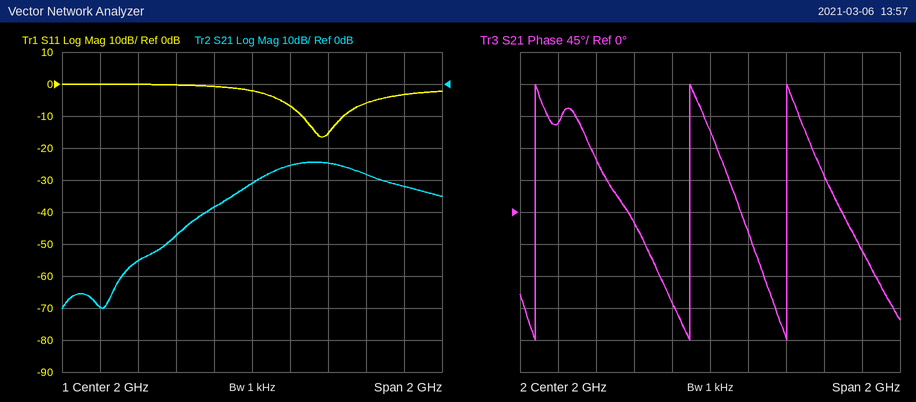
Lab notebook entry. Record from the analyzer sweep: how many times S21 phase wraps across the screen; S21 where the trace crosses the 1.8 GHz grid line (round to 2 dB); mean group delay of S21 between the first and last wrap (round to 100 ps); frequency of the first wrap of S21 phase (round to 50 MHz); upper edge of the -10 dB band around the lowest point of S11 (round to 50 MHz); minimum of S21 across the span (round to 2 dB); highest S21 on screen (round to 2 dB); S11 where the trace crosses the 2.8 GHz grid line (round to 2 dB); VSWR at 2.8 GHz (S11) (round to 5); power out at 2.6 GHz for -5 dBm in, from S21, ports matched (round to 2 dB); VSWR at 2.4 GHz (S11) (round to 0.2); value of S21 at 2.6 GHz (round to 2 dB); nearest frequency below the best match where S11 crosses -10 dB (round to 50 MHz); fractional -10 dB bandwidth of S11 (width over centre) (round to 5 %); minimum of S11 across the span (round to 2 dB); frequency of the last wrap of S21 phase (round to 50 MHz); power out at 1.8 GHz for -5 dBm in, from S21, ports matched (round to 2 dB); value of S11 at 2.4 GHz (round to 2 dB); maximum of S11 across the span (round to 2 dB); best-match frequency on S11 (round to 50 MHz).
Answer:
3
-38 dB
1.5 ns
1.10 GHz
2.50 GHz
-70 dB
-24 dB
-4 dB
5
-34 dBm
1.4
-28 dB
2.25 GHz
10 %
-16 dB
2.40 GHz
-44 dBm
-16 dB
0 dB
2.35 GHz
